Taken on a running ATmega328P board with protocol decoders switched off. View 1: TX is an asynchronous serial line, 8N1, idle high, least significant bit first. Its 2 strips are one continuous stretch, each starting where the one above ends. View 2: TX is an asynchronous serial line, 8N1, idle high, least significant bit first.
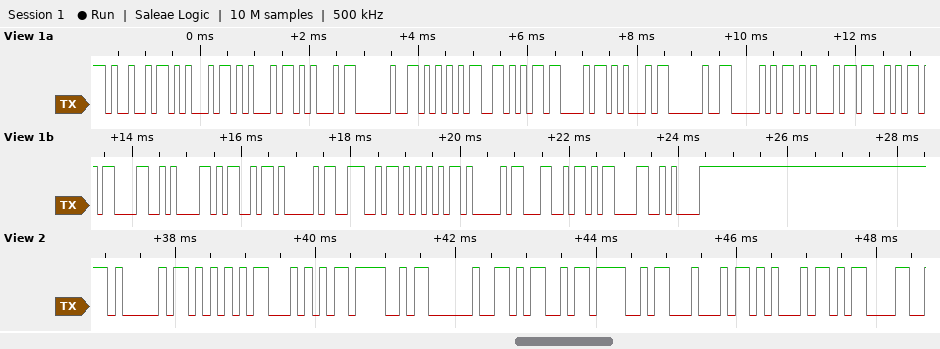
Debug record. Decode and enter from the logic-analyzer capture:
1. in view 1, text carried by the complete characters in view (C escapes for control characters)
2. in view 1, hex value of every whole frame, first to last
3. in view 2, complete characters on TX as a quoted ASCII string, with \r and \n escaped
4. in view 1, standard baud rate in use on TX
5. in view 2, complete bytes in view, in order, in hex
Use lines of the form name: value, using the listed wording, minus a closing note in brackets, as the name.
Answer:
in view 1, text carried by the complete characters in view: "IEEE UVCE PES\r\nMANUAL\r\n"
in view 1, hex value of every whole frame, first to last: 49 45 45 45 20 55 56 43 45 20 50 45 53 0D 0A 4D 41 4E 55 41 4C 0D 0A
in view 2, complete characters on TX as a quoted ASCII string, with \r and \n escaped: "AUTO MODE\r"
in view 1, standard baud rate in use on TX: 9600 baud
in view 2, complete bytes in view, in order, in hex: 0x41 0x55 0x54 0x4F 0x20 0x4D 0x4F 0x44 0x45 0x0D
